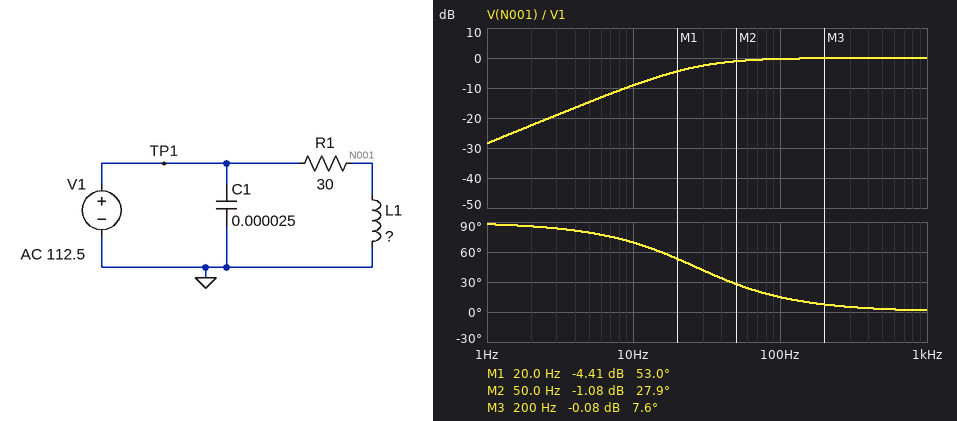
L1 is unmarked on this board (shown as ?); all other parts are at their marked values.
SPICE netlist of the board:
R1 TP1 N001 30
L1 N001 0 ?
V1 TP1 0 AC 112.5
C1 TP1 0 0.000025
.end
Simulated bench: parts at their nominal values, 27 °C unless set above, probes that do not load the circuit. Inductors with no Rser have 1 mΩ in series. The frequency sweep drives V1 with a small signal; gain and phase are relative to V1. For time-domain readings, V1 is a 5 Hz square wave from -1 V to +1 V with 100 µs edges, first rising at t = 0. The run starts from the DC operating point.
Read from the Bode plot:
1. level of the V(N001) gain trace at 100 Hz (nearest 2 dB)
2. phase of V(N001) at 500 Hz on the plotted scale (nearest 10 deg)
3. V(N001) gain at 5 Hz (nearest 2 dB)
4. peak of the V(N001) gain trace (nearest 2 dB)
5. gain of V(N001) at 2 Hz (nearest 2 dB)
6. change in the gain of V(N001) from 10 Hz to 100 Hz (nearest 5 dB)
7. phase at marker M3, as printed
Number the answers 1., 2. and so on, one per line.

1. 0 dB
2. 0 deg
3. -14 dB
4. 0 dB
5. -22 dB
6. 10 dB
7. 7.6 deg
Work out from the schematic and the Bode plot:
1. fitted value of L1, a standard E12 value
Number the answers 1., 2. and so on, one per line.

1. 180 mH
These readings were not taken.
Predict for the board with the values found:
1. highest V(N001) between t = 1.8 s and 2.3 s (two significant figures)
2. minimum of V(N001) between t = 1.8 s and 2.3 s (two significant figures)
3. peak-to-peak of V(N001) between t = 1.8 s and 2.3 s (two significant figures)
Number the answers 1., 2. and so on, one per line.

1. 2.0 V
2. -2.0 V
3. 4.0 V
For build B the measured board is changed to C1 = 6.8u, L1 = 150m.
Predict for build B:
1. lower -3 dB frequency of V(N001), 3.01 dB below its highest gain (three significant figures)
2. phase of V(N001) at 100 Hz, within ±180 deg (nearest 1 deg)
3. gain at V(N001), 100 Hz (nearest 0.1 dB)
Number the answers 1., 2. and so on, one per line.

1. 31.8 Hz
2. 18 deg
3. -0.4 dB
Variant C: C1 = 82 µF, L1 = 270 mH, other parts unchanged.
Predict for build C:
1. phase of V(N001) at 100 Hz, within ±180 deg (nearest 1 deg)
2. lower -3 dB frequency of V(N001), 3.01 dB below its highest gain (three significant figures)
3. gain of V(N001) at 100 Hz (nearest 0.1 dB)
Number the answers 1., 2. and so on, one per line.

1. 10 deg
2. 17.7 Hz
3. -0.1 dB
